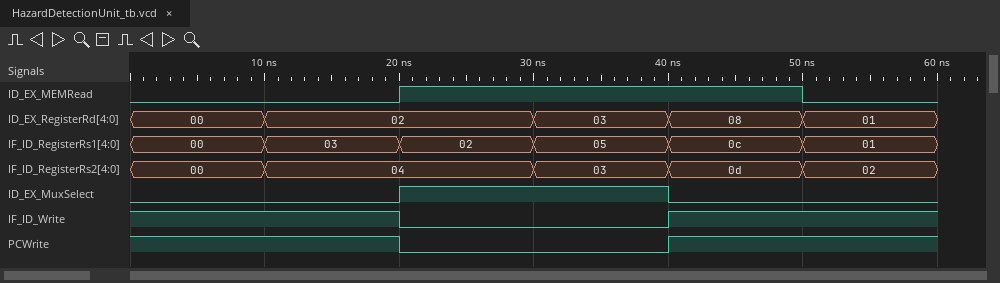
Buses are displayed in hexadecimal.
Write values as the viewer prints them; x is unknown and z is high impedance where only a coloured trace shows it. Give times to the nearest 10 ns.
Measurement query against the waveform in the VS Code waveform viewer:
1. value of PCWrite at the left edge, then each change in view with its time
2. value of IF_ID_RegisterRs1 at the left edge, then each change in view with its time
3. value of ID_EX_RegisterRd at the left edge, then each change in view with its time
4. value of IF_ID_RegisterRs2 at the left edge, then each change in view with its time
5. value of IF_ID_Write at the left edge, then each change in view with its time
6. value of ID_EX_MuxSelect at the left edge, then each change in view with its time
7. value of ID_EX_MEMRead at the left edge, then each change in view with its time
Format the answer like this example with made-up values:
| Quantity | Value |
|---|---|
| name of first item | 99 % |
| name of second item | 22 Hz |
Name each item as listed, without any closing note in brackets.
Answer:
| Quantity | Value |
|---|---|
| value of PCWrite at the left edge, then each change in view with its time | 1, 0 at 20 ns, 1 at 40 ns |
| value of IF_ID_RegisterRs1 at the left edge, then each change in view with its time | 00, 03 at 10 ns, 02 at 20 ns, 05 at 30 ns, 0c at 40 ns, 01 at 50 ns |
| value of ID_EX_RegisterRd at the left edge, then each change in view with its time | 00, 02 at 10 ns, 03 at 30 ns, 08 at 40 ns, 01 at 50 ns |
| value of IF_ID_RegisterRs2 at the left edge, then each change in view with its time | 00, 04 at 10 ns, 03 at 30 ns, 0d at 40 ns, 02 at 50 ns |
| value of IF_ID_Write at the left edge, then each change in view with its time | 1, 0 at 20 ns, 1 at 40 ns |
| value of ID_EX_MuxSelect at the left edge, then each change in view with its time | 0, 1 at 20 ns, 0 at 40 ns |
| value of ID_EX_MEMRead at the left edge, then each change in view with its time | 0, 1 at 20 ns, 0 at 50 ns |
